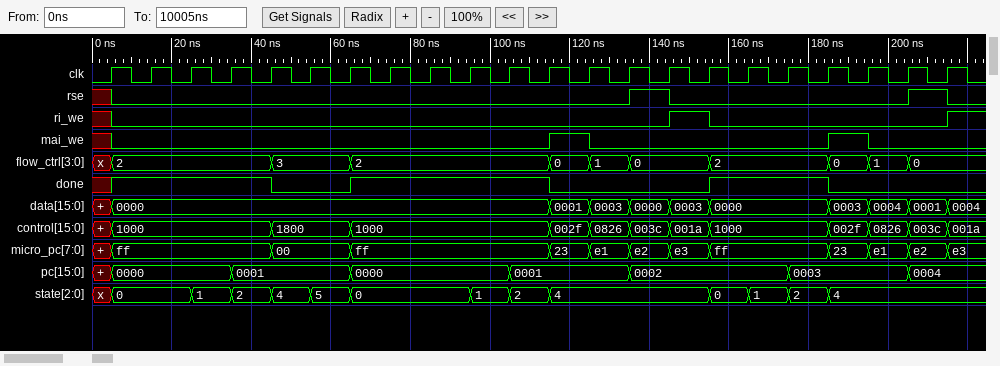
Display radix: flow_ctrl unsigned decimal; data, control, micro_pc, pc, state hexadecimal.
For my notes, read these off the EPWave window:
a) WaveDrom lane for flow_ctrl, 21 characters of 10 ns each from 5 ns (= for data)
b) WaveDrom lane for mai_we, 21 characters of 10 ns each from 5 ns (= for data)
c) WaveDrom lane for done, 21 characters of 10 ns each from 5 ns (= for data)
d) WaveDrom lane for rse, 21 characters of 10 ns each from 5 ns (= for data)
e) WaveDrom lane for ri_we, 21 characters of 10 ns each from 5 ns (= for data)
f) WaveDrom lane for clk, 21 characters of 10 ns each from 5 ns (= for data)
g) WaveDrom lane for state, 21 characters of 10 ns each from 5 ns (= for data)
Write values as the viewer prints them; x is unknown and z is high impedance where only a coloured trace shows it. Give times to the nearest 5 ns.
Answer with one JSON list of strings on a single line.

["{name: 'flow_ctrl', wave: '=...=.=....===.=..===', data: '2 3 2 0 1 0 2 0 1 0'}", "{name: 'mai_we', wave: '0..........10.....10.'}", "{name: 'done', wave: '1...0.1....0...1..0..'}", "{name: 'rse', wave: '0............10.....1'}", "{name: 'ri_we', wave: '0.............10.....'}", "{name: 'clk', wave: 'p....................'}", "{name: 'state', wave: '=.=====..===...====..', data: '0 1 2 4 5 0 1 2 4 0 1 2 4'}"]
